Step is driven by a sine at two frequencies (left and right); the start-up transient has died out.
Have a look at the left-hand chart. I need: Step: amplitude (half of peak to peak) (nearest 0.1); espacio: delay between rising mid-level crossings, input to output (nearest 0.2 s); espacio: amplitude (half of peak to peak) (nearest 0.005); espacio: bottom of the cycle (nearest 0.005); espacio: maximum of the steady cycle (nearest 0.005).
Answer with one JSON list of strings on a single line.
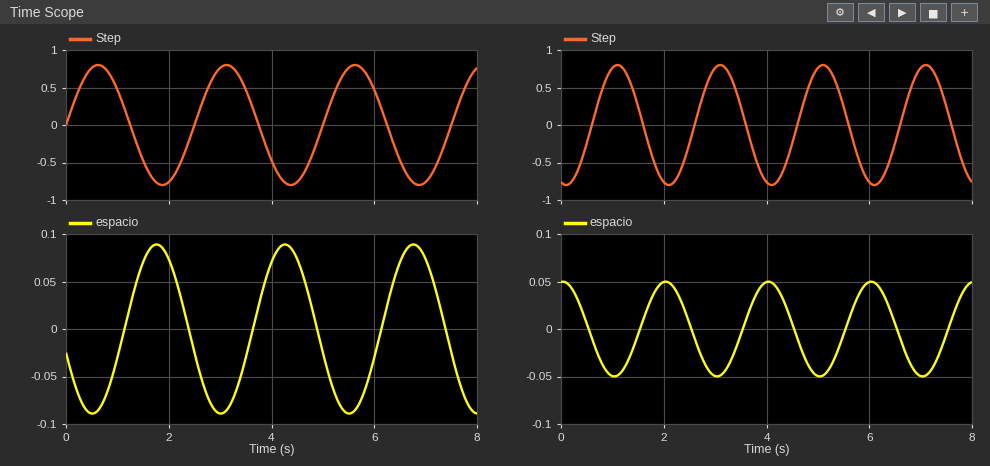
["0.8", "1.2 s", "0.090", "-0.090", "0.090"]
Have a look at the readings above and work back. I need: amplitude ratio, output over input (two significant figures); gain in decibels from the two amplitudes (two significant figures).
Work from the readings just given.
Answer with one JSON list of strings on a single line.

["0.11", "-19 dB"]
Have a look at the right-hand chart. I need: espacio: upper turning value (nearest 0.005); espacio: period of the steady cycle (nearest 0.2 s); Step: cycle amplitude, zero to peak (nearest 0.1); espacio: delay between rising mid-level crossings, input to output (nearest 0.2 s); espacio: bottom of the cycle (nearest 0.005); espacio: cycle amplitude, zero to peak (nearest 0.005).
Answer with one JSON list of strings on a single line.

["0.050", "2.0 s", "0.8", "1.0 s", "-0.050", "0.050"]
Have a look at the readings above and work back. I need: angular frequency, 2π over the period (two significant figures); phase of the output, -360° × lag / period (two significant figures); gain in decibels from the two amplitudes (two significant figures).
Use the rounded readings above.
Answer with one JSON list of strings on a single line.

["3.1 rad/s", "-180°", "-24 dB"]
